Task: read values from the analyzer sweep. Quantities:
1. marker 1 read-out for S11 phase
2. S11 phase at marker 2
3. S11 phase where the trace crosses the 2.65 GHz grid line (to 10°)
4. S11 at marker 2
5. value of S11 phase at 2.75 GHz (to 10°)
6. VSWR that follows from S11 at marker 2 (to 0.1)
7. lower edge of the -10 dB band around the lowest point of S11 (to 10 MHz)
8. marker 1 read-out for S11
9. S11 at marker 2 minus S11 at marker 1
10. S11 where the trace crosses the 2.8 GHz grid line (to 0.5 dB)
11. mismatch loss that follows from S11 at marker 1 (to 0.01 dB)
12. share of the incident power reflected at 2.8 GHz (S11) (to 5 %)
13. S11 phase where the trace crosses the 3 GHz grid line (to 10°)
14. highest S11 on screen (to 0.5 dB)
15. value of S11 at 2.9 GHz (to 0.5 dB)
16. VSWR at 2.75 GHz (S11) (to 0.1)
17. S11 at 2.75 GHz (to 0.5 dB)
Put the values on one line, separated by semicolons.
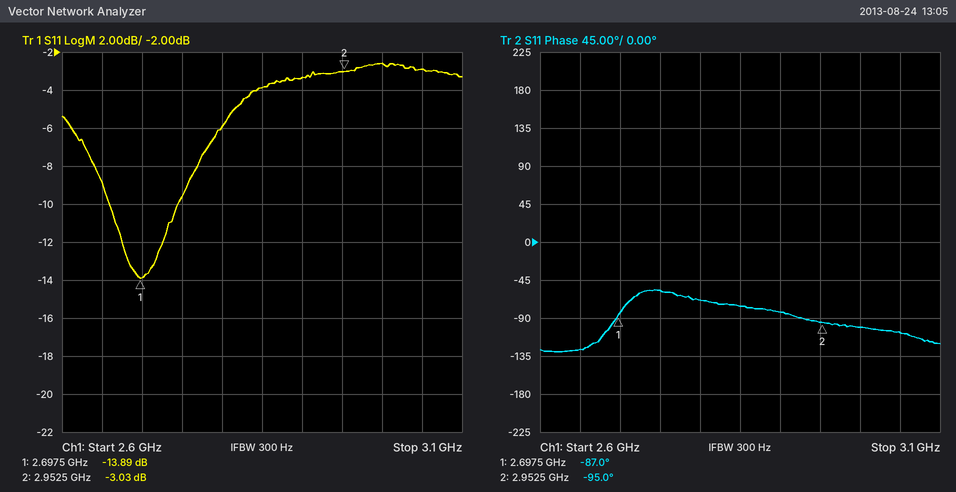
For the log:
-87.0°; -95.0°; -130°; -3.03 dB; -60°; 5.8; 2.66 GHz; -13.89 dB; 10.86 dB; -6.0 dB; 0.18 dB; 25 %; -100°; -2.5 dB; -3.5 dB; 2.0; -9.5 dB
